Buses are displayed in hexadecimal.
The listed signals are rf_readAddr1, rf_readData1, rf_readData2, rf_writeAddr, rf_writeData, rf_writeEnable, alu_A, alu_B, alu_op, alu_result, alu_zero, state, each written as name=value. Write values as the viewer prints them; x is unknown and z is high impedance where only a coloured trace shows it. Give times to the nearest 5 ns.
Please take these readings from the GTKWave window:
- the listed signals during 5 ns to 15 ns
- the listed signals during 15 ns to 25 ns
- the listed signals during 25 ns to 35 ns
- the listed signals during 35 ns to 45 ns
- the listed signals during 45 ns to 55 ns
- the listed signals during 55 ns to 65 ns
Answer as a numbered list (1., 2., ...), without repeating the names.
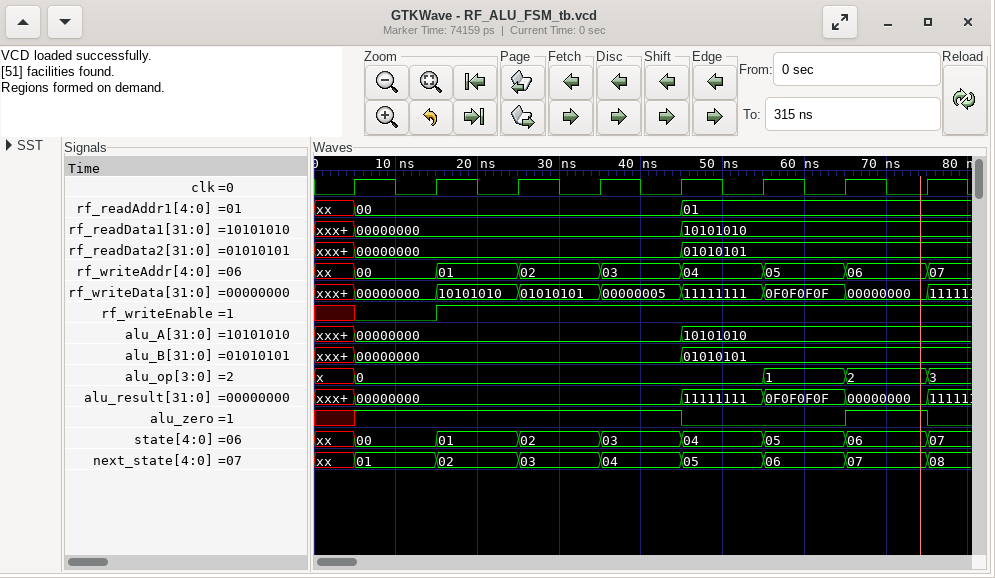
1. rf_readAddr1=00, rf_readData1=00000000, rf_readData2=00000000, rf_writeAddr=00, rf_writeData=00000000, rf_writeEnable=0, alu_A=00000000, alu_B=00000000, alu_op=0, alu_result=00000000, alu_zero=1, state=00
2. rf_readAddr1=00, rf_readData1=00000000, rf_readData2=00000000, rf_writeAddr=01, rf_writeData=10101010, rf_writeEnable=1, alu_A=00000000, alu_B=00000000, alu_op=0, alu_result=00000000, alu_zero=1, state=01
3. rf_readAddr1=00, rf_readData1=00000000, rf_readData2=00000000, rf_writeAddr=02, rf_writeData=01010101, rf_writeEnable=1, alu_A=00000000, alu_B=00000000, alu_op=0, alu_result=00000000, alu_zero=1, state=02
4. rf_readAddr1=00, rf_readData1=00000000, rf_readData2=00000000, rf_writeAddr=03, rf_writeData=00000005, rf_writeEnable=1, alu_A=00000000, alu_B=00000000, alu_op=0, alu_result=00000000, alu_zero=1, state=03
5. rf_readAddr1=01, rf_readData1=10101010, rf_readData2=01010101, rf_writeAddr=04, rf_writeData=11111111, rf_writeEnable=1, alu_A=10101010, alu_B=01010101, alu_op=0, alu_result=11111111, alu_zero=0, state=04
6. rf_readAddr1=01, rf_readData1=10101010, rf_readData2=01010101, rf_writeAddr=05, rf_writeData=0F0F0F0F, rf_writeEnable=1, alu_A=10101010, alu_B=01010101, alu_op=1, alu_result=0F0F0F0F, alu_zero=0, state=05
